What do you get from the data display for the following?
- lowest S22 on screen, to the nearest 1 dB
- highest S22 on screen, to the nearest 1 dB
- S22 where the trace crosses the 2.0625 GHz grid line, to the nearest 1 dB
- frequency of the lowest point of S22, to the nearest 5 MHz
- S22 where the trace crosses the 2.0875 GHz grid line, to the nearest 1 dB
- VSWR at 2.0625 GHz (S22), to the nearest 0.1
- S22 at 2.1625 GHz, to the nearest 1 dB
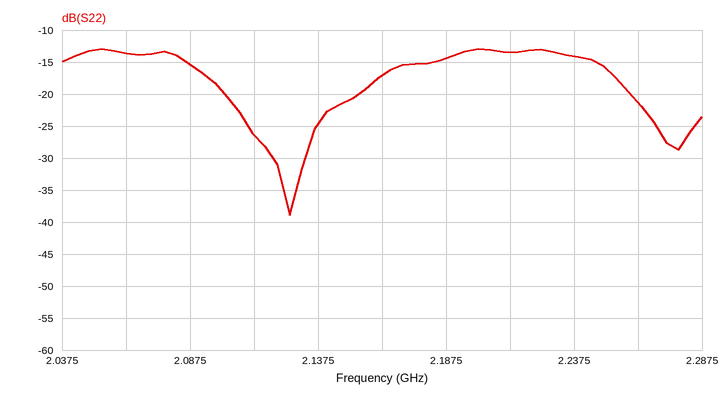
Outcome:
-39 dB
-13 dB
-14 dB
2.125 GHz
-15 dB
1.5
-17 dB
